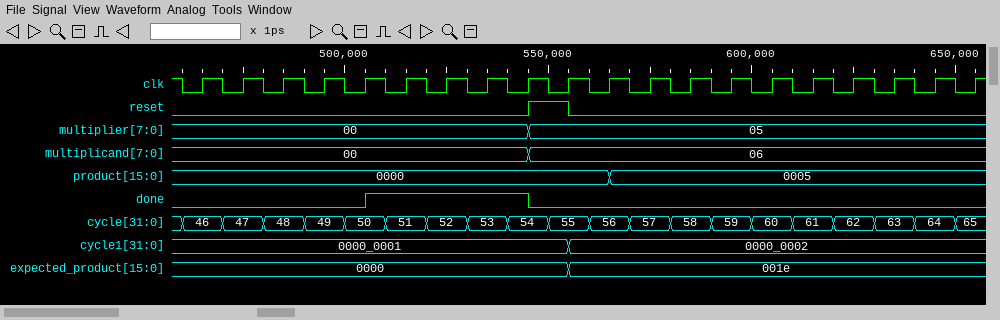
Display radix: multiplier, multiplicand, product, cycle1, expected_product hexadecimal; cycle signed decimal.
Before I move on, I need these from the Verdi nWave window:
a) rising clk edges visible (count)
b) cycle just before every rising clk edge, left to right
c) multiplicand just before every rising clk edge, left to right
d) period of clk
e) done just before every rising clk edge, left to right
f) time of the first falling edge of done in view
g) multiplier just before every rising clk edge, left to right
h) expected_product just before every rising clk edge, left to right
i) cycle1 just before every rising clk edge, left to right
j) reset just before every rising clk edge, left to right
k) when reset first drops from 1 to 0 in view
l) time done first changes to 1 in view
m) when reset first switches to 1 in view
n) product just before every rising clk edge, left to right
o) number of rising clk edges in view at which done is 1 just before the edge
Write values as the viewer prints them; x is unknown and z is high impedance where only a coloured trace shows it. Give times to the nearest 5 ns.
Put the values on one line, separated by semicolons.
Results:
20; 46, 47, 48, 49, 50, 51, 52, 53, 54, 55, 56, 57, 58, 59, 60, 61, 62, 63, 64, 65; 00, 00, 00, 00, 00, 00, 00, 00, 00, 06, 06, 06, 06, 06, 06, 06, 06, 06, 06, 06; 10 ns; 0 0 0 0 0 1 1 1 1 0 0 0 0 0 0 0 0 0 0 0; 545 ns; 00, 00, 00, 00, 00, 00, 00, 00, 00, 05, 05, 05, 05, 05, 05, 05, 05, 05, 05, 05; 0000, 0000, 0000, 0000, 0000, 0000, 0000, 0000, 0000, 0000, 001e, 001e, 001e, 001e, 001e, 001e, 001e, 001e, 001e, 001e; 0000_0001, 0000_0001, 0000_0001, 0000_0001, 0000_0001, 0000_0001, 0000_0001, 0000_0001, 0000_0001, 0000_0001, 0000_0002, 0000_0002, 0000_0002, 0000_0002, 0000_0002, 0000_0002, 0000_0002, 0000_0002, 0000_0002, 0000_0002; 0 0 0 0 0 0 0 0 0 1 0 0 0 0 0 0 0 0 0 0; 555 ns; 505 ns; 545 ns; 0000, 0000, 0000, 0000, 0000, 0000, 0000, 0000, 0000, 0000, 0000, 0005, 0005, 0005, 0005, 0005, 0005, 0005, 0005, 0005; 4
